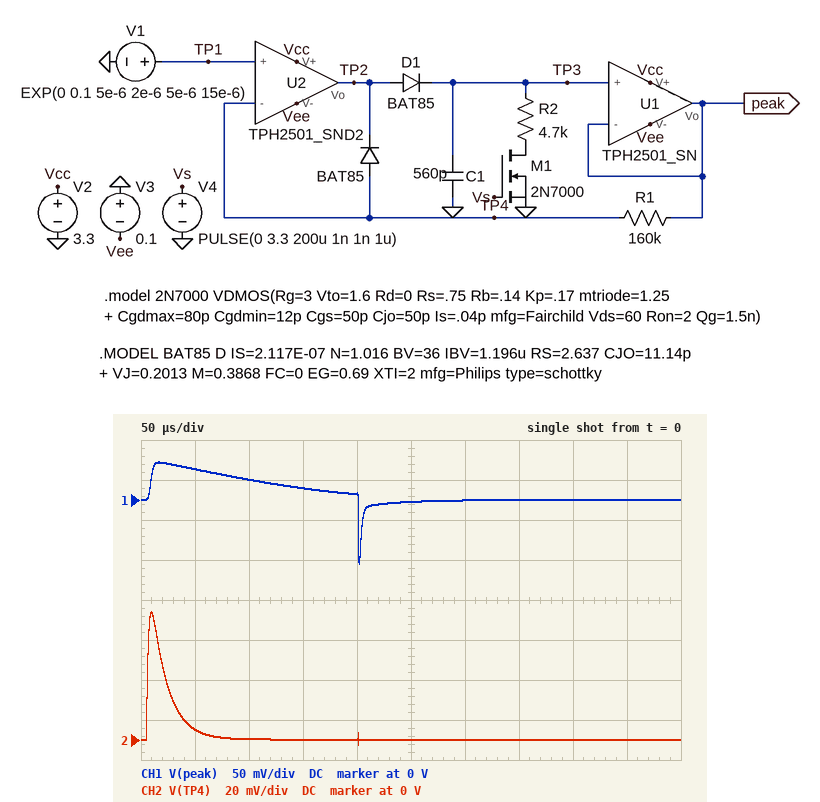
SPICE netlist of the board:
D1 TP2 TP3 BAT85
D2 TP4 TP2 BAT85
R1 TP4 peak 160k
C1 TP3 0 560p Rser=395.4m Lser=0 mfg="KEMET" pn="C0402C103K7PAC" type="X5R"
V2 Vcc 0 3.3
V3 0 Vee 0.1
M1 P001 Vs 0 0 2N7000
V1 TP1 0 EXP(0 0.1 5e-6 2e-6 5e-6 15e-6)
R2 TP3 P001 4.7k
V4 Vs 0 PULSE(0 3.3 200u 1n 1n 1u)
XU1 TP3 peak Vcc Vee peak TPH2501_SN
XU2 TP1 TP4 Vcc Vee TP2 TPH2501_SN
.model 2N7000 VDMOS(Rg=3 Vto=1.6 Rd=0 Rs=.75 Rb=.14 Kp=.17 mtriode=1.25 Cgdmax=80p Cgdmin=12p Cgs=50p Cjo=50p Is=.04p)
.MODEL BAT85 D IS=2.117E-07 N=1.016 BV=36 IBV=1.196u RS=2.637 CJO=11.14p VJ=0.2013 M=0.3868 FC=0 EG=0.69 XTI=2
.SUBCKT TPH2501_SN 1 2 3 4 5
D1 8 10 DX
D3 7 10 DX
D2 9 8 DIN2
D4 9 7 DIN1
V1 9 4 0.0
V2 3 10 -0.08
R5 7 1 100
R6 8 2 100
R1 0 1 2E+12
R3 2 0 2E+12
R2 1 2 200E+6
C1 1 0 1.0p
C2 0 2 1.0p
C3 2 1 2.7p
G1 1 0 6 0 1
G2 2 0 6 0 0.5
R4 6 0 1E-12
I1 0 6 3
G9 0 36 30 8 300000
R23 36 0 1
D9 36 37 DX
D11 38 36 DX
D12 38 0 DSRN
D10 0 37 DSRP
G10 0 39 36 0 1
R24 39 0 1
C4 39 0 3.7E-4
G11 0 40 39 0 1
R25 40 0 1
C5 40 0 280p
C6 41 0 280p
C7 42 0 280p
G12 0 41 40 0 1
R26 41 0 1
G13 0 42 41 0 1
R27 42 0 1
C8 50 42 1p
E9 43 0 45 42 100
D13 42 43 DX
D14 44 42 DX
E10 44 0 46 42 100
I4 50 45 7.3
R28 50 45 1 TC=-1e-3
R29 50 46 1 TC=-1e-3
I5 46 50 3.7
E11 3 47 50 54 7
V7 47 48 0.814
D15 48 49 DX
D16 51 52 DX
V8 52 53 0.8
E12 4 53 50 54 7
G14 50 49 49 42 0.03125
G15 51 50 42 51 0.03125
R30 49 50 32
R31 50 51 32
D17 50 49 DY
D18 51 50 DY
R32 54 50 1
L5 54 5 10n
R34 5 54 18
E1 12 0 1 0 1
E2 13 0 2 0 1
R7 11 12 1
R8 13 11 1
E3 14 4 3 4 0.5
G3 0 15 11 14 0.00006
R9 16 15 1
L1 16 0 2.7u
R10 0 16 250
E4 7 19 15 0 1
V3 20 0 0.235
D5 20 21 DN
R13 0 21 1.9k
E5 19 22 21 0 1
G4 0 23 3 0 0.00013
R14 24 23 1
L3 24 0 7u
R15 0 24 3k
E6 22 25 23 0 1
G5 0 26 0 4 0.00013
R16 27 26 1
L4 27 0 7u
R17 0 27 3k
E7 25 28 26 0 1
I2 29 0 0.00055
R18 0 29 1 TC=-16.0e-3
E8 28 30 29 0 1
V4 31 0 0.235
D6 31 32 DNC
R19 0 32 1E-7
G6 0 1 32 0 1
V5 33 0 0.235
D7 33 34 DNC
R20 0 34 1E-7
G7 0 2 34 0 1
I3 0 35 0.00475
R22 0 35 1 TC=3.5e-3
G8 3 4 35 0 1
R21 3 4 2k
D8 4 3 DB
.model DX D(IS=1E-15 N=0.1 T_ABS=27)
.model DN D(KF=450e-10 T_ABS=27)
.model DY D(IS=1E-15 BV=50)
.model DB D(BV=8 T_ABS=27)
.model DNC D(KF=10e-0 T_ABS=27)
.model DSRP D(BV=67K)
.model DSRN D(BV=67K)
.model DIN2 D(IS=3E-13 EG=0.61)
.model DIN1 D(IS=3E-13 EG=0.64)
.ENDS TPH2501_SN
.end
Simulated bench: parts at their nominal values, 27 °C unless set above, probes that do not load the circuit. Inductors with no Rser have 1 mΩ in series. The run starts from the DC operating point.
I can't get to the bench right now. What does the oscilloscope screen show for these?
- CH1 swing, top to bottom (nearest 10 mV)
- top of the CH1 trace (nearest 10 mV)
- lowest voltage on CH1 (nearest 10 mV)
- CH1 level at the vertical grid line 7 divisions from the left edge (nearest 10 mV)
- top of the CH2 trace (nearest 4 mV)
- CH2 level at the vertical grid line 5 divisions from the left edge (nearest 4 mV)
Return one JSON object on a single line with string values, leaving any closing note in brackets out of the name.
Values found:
{"CH1 swing, top to bottom": "130 mV", "top of the CH1 trace": "50 mV", "lowest voltage on CH1": "-80 mV", "CH1 level at the vertical grid line 7 divisions from the left edge": "0 V", "top of the CH2 trace": "64 mV", "CH2 level at the vertical grid line 5 divisions from the left edge": "0 V"}
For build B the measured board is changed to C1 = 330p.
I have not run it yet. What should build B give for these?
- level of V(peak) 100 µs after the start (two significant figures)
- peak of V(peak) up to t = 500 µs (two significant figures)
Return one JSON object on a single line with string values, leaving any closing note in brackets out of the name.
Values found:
{"level of V(peak) 100 µs after the start": "18 mV", "peak of V(peak) up to t = 500 µs": "49 mV"}
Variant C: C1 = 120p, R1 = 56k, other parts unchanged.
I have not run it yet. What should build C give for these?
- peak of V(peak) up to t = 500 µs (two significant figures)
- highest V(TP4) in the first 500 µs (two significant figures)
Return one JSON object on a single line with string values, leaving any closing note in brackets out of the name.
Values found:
{"peak of V(peak) up to t = 500 µs": "66 mV", "highest V(TP4) in the first 500 µs": "64 mV"}
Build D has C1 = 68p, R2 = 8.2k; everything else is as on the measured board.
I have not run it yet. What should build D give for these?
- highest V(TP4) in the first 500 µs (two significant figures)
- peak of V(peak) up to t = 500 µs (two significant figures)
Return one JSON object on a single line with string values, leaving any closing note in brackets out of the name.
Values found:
{"highest V(TP4) in the first 500 µs": "64 mV", "peak of V(peak) up to t = 500 µs": "52 mV"}
